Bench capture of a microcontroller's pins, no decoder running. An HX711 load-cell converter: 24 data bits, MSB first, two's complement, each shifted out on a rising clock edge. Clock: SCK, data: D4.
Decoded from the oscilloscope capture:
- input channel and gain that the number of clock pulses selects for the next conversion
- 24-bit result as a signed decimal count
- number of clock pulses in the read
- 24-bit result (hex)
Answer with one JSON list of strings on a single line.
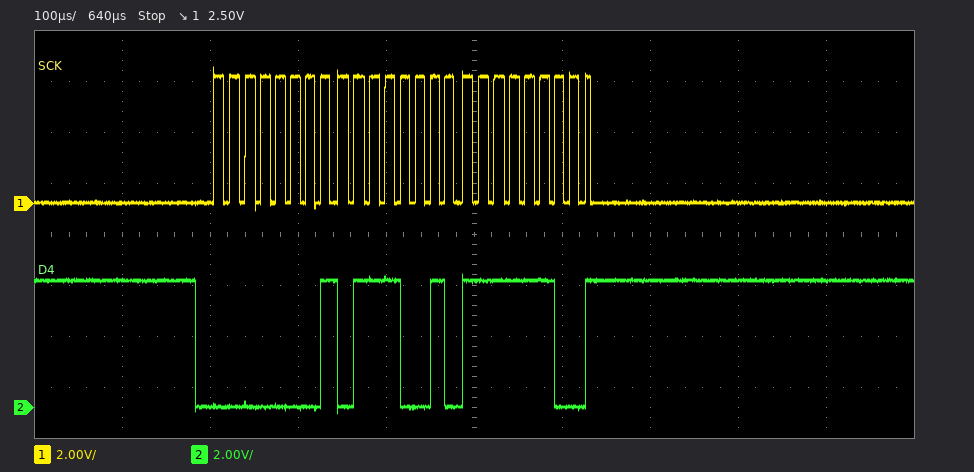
["channel A, gain 128", "94972", "25", "0x0172FC"]
